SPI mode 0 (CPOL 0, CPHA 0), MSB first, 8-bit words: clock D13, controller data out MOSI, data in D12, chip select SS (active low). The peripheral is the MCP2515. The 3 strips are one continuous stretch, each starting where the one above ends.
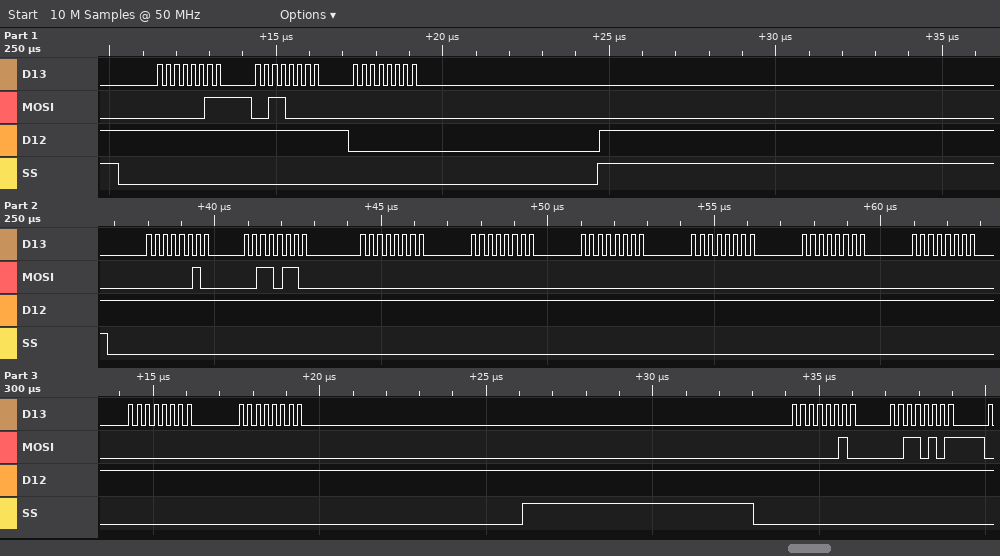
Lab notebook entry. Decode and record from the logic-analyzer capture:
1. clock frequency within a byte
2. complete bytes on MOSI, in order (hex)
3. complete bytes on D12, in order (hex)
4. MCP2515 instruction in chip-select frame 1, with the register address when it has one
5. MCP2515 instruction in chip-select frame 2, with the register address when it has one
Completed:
4 MHz
0x03 0x30 0x00 0x02 0x36 0x00 0x00 0x00 0x00 0x00 0x00 0x00 0x00 0x02 0x35
0xFF 0xFF 0x00 0xFF 0xFF 0xFF 0xFF 0xFF 0xFF 0xFF 0xFF 0xFF 0xFF 0xFF 0xFF
READ 0x30
WRITE 0x36
